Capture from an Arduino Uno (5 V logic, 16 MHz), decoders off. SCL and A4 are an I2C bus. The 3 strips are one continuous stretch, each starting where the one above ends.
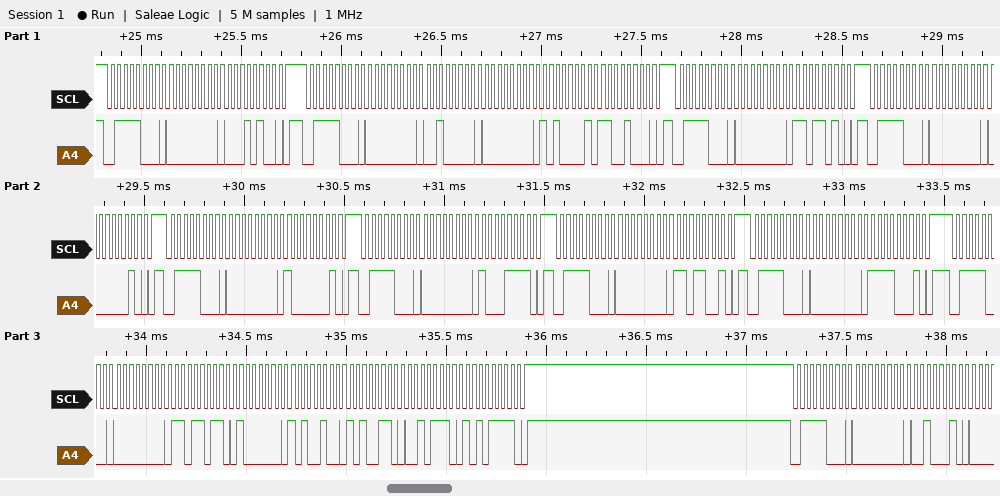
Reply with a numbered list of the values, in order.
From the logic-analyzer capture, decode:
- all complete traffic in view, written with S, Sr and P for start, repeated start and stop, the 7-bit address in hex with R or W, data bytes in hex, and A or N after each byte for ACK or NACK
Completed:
1. S 3CW A 00 A 14 A P S 3CW A 00 A 20 A 00 A A1 A C8 A P S 3CW A 00 A DA A P S 3CW A 00 A 02 A P S 3CW A 00 A 81 A P S 3CW A 00 A 8F A P S 3CW A 00 A D9 A P S 3CW A 00 A F1 A P S 3CW A 00 A DB A 40 A A4 A A6 A 2E A AF A P S 3CW A 00 A 22 A
